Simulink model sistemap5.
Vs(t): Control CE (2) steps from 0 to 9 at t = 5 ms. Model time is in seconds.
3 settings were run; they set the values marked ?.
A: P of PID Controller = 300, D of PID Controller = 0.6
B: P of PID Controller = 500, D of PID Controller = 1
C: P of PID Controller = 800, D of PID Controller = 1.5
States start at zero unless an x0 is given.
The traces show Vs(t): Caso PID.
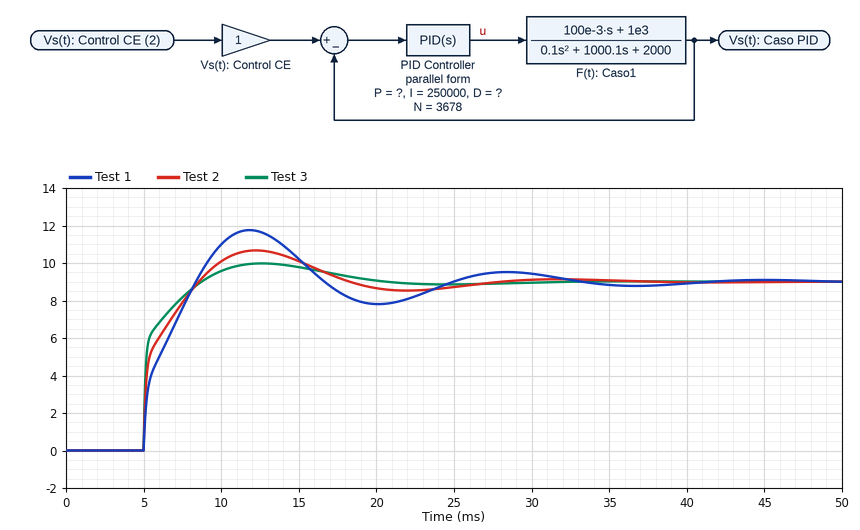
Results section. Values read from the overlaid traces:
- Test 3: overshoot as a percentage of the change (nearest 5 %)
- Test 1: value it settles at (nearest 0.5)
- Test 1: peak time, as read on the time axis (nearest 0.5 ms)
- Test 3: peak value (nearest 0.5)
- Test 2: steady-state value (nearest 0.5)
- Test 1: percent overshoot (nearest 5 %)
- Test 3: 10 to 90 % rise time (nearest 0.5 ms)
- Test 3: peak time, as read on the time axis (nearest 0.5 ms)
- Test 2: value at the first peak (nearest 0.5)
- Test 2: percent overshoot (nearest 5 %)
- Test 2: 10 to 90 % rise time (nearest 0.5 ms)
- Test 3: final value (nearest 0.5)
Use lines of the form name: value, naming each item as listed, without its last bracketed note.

Test 3: overshoot as a percentage of the change: 10 %
Test 1: value it settles at: 9.0
Test 1: peak time, as read on the time axis: 12.0 ms
Test 3: peak value: 10.0
Test 2: steady-state value: 9.0
Test 1: percent overshoot: 30 %
Test 3: 10 to 90 % rise time: 2.5 ms
Test 3: peak time, as read on the time axis: 12.5 ms
Test 2: value at the first peak: 10.5
Test 2: percent overshoot: 20 %
Test 2: 10 to 90 % rise time: 2.5 ms
Test 3: final value: 9.0
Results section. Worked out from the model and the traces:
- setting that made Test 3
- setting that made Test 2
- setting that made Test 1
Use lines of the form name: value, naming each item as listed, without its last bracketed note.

setting that made Test 3: C
setting that made Test 2: B
setting that made Test 1: A
